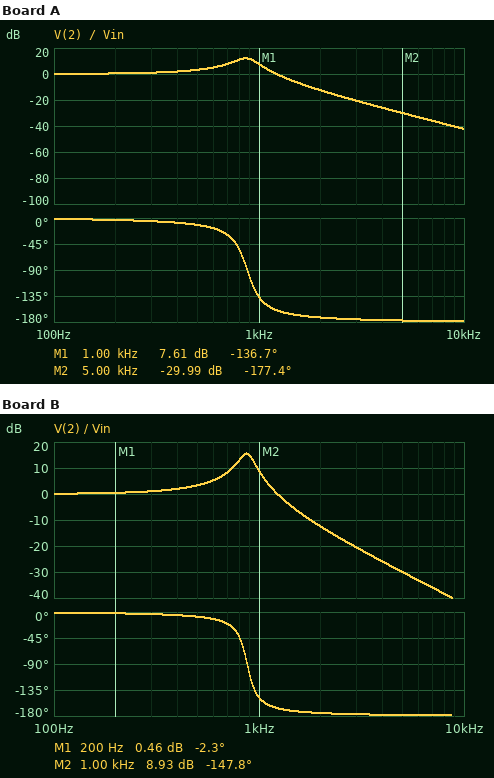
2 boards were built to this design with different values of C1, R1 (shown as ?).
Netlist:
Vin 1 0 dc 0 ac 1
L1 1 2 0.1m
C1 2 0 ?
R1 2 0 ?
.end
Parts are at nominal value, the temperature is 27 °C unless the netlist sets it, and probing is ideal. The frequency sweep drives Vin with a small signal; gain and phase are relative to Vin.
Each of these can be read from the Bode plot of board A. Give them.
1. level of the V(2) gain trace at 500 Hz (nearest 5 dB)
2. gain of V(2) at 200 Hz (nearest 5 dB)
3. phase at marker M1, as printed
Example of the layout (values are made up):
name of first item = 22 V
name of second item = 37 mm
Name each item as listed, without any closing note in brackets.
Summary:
level of the V(2) gain trace at 500 Hz = 5 dB
gain of V(2) at 200 Hz = 0 dB
phase at marker M1, as printed = -136.7 deg
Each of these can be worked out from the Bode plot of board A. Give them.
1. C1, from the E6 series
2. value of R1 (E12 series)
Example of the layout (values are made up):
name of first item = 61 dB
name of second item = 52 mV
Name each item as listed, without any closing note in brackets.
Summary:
C1, from the E6 series = 330 µF
value of R1 = 2.2 Ω
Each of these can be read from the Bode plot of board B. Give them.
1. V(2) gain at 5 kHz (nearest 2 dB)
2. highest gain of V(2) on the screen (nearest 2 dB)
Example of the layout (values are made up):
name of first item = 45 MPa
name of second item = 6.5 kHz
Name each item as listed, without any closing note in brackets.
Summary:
V(2) gain at 5 kHz = -30 dB
highest gain of V(2) on the screen = 16 dB
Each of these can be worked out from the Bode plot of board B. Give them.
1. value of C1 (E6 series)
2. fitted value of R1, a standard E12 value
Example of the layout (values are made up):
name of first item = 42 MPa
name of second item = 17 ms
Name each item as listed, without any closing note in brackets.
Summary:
value of C1 = 330 µF
fitted value of R1, a standard E12 value = 3.3 Ω
